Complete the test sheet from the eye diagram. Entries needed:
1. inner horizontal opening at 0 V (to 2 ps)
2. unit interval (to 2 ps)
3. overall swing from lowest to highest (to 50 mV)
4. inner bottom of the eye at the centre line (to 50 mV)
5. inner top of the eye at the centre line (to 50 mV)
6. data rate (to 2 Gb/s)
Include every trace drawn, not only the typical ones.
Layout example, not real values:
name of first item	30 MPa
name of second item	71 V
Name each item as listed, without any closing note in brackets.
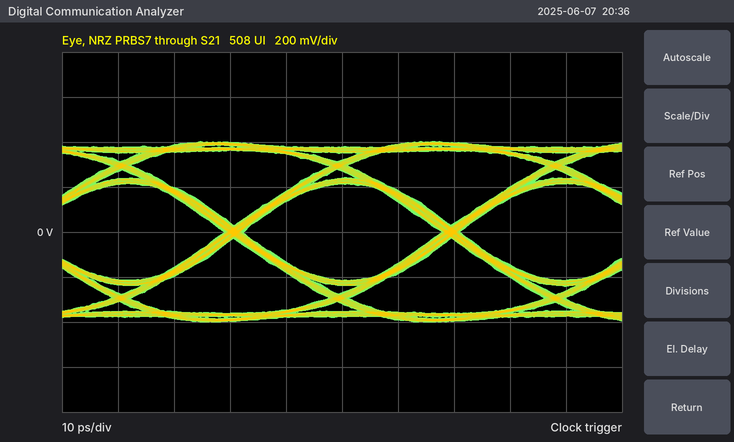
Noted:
inner horizontal opening at 0 V	36 ps
unit interval	38 ps
overall swing from lowest to highest	800 mV
inner bottom of the eye at the centre line	-200 mV
inner top of the eye at the centre line	200 mV
data rate	26 Gb/s
